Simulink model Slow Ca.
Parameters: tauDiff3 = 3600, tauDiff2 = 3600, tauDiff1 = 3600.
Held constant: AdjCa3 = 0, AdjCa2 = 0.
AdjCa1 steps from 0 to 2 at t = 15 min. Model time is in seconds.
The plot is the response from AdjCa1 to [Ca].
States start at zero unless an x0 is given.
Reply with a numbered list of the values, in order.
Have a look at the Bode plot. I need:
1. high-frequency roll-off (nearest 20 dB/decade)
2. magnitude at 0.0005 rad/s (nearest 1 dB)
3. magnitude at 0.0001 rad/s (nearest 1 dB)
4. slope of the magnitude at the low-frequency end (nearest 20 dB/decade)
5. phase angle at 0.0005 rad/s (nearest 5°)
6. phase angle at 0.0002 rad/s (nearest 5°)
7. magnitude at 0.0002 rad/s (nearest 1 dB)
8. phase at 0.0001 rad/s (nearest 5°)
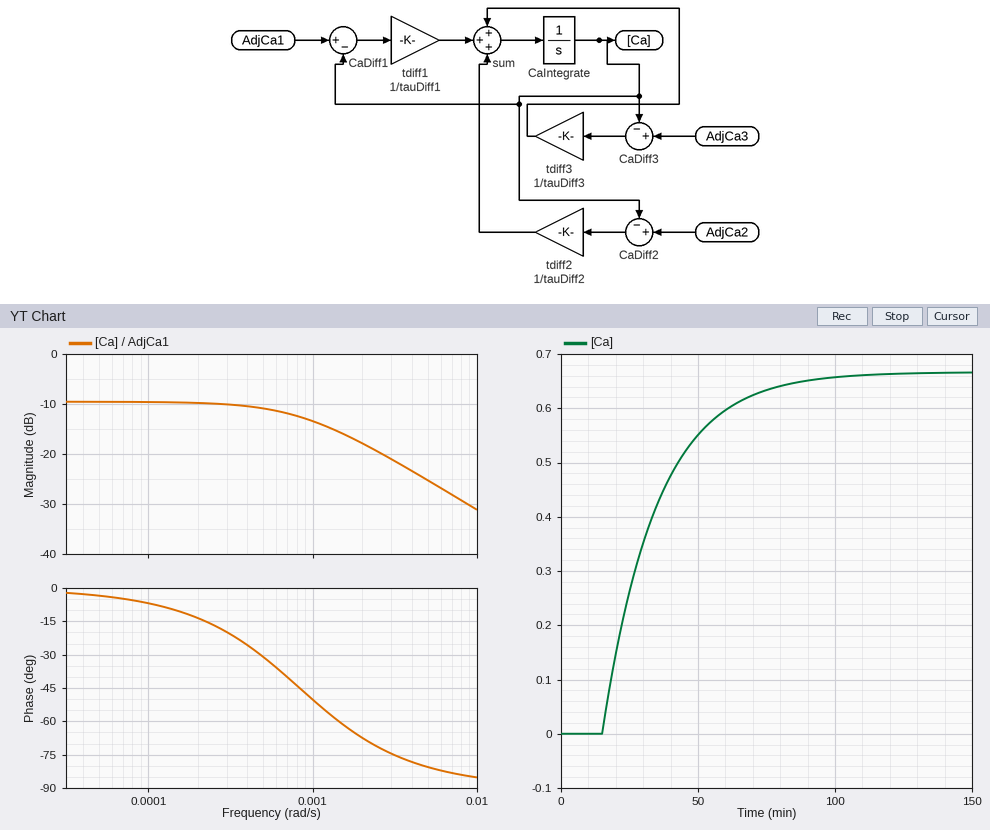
1. -20 dB/decade
2. -11 dB
3. -10 dB
4. 0 dB/decade
5. -30°
6. -15°
7. -10 dB
8. -5°
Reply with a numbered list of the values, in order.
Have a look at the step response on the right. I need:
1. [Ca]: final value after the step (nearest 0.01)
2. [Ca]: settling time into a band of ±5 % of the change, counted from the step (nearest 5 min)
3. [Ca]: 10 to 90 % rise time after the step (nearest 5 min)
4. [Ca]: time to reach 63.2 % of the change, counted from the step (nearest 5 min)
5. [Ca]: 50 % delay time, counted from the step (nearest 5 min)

1. 0.67
2. 60 min
3. 45 min
4. 20 min
5. 15 min
